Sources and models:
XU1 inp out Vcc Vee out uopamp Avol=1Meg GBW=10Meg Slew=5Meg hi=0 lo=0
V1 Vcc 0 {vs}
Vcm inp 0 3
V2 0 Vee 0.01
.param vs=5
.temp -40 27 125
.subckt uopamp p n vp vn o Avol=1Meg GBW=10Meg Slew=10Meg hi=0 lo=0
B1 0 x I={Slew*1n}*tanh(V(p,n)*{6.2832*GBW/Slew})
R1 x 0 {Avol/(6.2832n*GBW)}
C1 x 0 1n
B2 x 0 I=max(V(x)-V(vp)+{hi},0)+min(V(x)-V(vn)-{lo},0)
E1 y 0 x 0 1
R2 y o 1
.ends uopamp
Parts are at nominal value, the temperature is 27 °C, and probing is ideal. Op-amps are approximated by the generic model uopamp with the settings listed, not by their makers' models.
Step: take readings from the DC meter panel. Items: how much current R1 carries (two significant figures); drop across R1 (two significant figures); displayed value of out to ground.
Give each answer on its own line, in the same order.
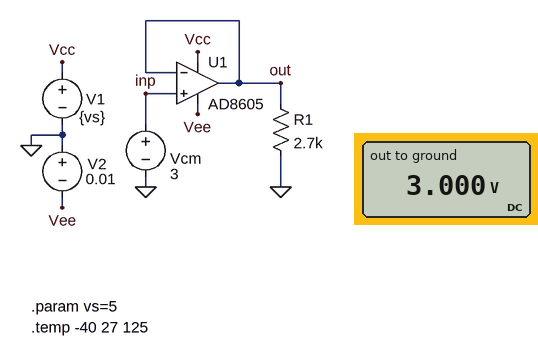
1.1 mA
3.0 V
3.000 V
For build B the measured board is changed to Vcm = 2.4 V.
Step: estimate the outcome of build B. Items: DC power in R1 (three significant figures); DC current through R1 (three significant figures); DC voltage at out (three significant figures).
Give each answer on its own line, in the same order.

2.13 mW
889 µA
2.40 V
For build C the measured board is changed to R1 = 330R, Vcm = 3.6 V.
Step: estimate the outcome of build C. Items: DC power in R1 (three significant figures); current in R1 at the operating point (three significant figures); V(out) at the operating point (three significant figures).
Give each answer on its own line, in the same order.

39.3 mW
10.9 mA
3.60 V
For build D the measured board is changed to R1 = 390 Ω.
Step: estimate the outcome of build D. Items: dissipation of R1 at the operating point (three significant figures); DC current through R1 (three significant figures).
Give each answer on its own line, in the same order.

23.1 mW
7.69 mA
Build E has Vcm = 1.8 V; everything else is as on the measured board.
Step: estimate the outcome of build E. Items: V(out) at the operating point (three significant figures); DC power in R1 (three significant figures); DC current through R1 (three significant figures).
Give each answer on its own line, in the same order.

1.80 V
1.20 mW
667 µA
